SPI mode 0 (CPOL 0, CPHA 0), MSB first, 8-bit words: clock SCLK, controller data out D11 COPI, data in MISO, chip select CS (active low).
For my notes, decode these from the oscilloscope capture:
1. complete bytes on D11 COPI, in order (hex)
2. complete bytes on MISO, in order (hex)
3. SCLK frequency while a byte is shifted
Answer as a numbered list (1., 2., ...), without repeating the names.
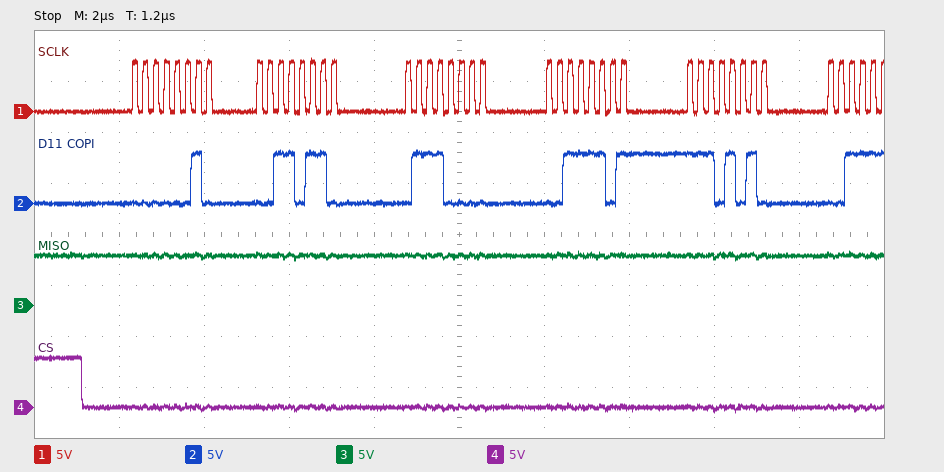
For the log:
1. 02 36 70 3D EA
2. FF FF FF FF FF
3. 4 MHz
